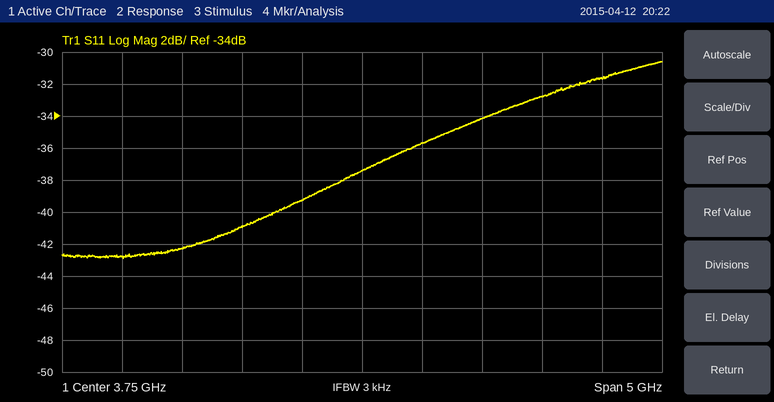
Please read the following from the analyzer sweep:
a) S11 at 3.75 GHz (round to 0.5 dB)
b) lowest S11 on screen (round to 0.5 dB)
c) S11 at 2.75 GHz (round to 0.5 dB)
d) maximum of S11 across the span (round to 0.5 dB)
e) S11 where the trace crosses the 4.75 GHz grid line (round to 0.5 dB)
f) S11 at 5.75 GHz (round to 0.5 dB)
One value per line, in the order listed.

-37.5 dB
-43.0 dB
-41.0 dB
-30.5 dB
-34.0 dB
-31.5 dB
